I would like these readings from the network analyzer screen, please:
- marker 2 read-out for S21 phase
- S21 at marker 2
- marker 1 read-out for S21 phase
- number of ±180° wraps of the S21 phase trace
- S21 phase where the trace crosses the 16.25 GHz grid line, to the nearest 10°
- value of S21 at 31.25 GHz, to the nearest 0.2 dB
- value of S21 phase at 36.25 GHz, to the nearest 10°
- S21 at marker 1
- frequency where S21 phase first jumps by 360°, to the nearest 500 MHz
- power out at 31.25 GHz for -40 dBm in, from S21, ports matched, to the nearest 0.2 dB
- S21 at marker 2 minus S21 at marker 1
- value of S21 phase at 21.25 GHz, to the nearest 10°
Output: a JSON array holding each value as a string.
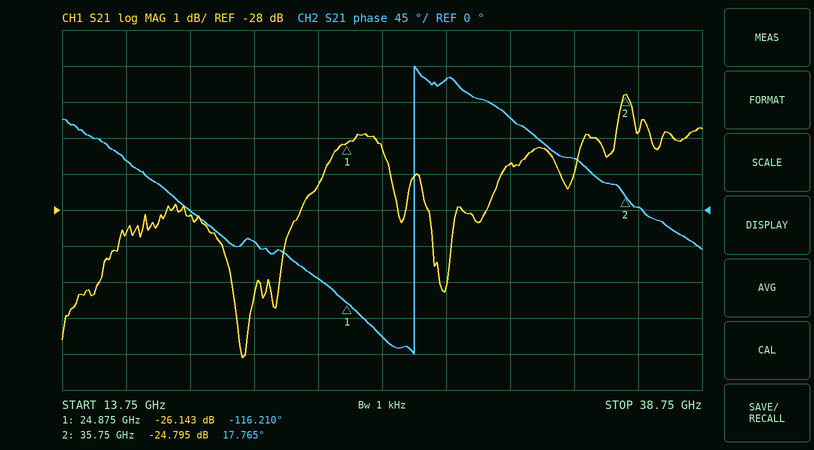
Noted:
["17.765°", "-24.795 dB", "-116.210°", "1", "60°", "-26.8 dB", "0°", "-26.143 dB", "27.5 GHz", "-66.8 dBm", "1.348 dB", "-40°"]
